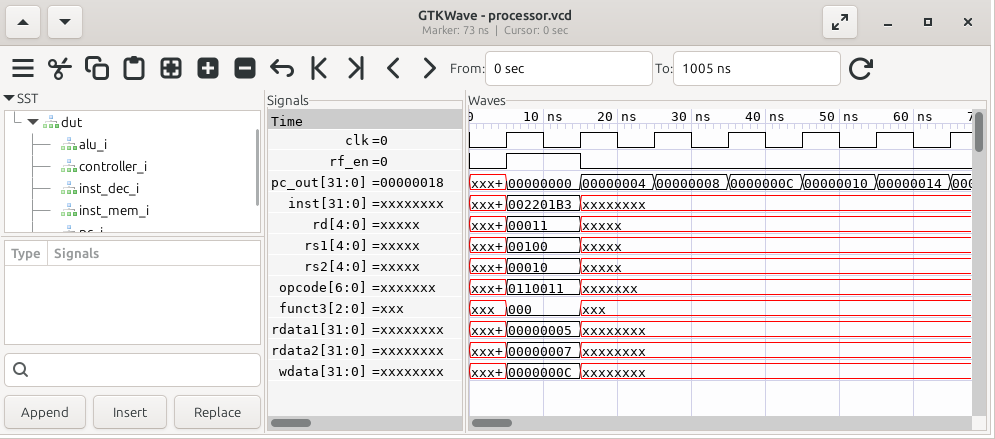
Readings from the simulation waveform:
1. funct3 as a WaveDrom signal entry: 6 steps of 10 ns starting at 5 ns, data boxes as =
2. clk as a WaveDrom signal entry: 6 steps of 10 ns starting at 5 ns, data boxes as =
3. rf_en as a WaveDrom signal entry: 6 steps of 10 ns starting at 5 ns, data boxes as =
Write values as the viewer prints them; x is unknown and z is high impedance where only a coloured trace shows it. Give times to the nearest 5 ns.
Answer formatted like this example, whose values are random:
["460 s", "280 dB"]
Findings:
["{name: 'funct3', wave: '=x....', data: '000'}", "{name: 'clk', wave: 'p.....'}", "{name: 'rf_en', wave: '10....'}"]
